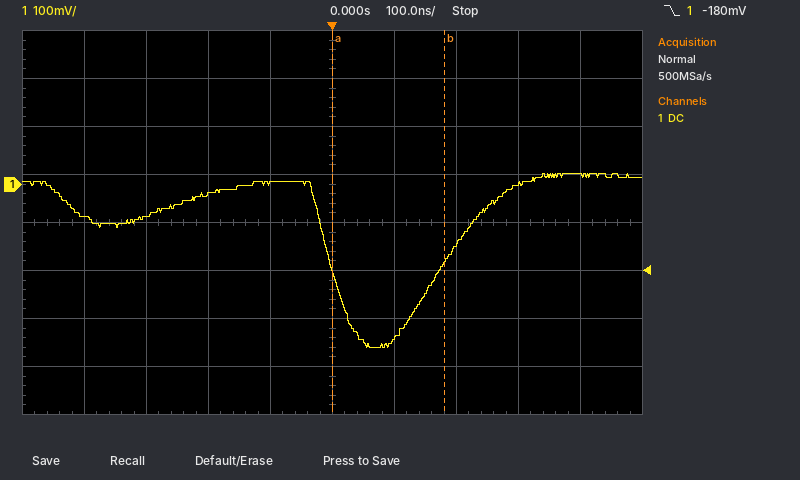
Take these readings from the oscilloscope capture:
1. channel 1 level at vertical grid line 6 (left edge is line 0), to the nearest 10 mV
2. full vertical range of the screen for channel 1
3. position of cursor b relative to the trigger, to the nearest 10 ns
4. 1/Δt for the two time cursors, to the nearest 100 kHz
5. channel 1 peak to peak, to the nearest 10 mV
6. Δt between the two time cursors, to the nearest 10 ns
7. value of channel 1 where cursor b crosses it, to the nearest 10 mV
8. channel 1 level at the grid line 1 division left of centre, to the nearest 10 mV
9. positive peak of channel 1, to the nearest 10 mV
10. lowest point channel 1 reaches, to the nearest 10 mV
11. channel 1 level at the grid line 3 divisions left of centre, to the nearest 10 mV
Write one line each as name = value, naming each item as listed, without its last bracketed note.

channel 1 level at vertical grid line 6 (left edge is line 0), to the nearest 10 mV = -320 mV
full vertical range of the screen for channel 1 = 800 mV
position of cursor b relative to the trigger, to the nearest 10 ns = +180 ns
1/Δt for the two time cursors, to the nearest 100 kHz = 5.6 MHz
channel 1 peak to peak, to the nearest 10 mV = 360 mV
Δt between the two time cursors, to the nearest 10 ns = 180 ns
value of channel 1 where cursor b crosses it, to the nearest 10 mV = -160 mV
channel 1 level at the grid line 1 division left of centre, to the nearest 10 mV = 0 mV
positive peak of channel 1, to the nearest 10 mV = 20 mV
lowest point channel 1 reaches, to the nearest 10 mV = -340 mV
channel 1 level at the grid line 3 divisions left of centre, to the nearest 10 mV = -70 mV
